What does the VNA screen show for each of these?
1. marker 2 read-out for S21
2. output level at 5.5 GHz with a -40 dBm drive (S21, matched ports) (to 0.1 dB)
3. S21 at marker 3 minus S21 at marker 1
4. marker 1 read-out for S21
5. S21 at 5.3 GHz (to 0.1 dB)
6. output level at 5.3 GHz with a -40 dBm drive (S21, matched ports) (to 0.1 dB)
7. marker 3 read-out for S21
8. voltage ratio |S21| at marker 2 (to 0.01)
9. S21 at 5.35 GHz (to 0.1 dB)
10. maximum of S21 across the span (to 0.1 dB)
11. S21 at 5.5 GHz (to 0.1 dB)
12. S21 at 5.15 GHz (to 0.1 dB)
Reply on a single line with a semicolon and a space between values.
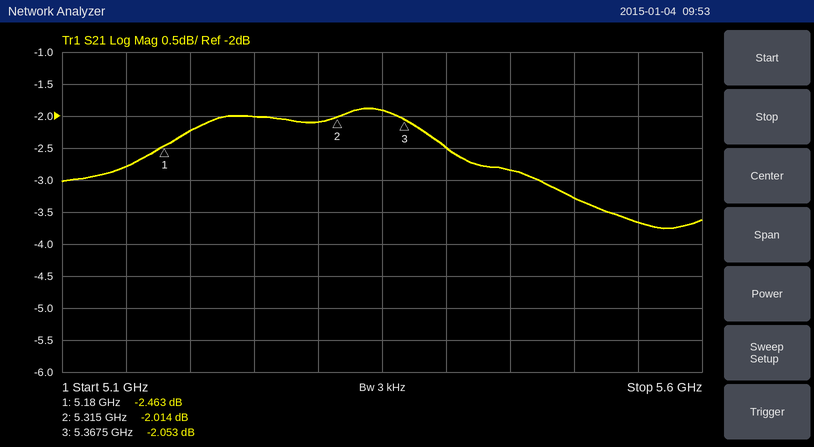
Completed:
-2.014 dB; -43.3 dBm; 0.410 dB; -2.463 dB; -2.1 dB; -42.1 dBm; -2.053 dB; 0.79; -1.9 dB; -1.9 dB; -3.3 dB; -2.8 dB
